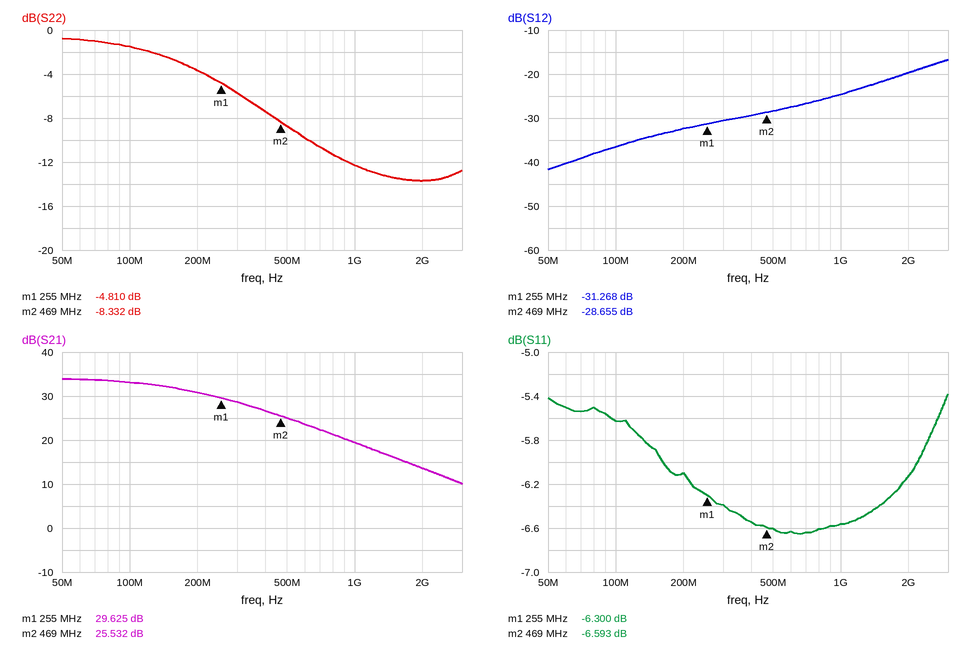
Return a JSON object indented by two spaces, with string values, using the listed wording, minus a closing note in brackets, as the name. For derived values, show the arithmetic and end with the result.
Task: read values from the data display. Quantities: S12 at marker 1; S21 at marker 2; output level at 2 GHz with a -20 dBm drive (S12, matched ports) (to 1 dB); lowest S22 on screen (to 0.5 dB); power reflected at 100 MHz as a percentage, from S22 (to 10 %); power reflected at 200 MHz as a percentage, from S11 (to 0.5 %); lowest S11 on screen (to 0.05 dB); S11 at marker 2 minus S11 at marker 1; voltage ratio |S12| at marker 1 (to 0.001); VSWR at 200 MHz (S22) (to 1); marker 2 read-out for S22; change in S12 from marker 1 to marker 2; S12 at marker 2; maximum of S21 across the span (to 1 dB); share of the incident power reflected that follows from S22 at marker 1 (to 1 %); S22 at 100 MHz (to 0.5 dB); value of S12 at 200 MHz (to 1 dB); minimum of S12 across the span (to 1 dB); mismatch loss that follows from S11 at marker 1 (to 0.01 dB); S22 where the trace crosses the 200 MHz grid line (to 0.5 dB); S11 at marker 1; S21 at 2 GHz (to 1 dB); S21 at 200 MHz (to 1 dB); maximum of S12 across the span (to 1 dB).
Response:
{
  "S12 at marker 1": "-31.268 dB",
  "S21 at marker 2": "25.532 dB",
  "output level at 2 GHz with a -20 dBm drive (S12, matched ports)": "-20 dBm + (-20 dB) = -40 dBm",
  "lowest S22 on screen": "-13.5 dB",
  "power reflected at 100 MHz as a percentage, from S22": "10^(-1.5/10) ≈ 70.8 %, so 70 % to the nearest 10 %",
  "power reflected at 200 MHz as a percentage, from S11": "10^(-6.1/10) ≈ 24.5 %",
  "lowest S11 on screen": "-6.65 dB",
  "S11 at marker 2 minus S11 at marker 1": "-6.593 − (-6.3) = -0.293 dB",
  "voltage ratio |S12| at marker 1": "10^(-31.268/20) ≈ 0.027",
  "VSWR at 200 MHz (S22)": "|Γ| = 10^(-3.5/20) = 0.6683; VSWR = (1 + 0.6683)/(1 − 0.6683) ≈ 5",
  "marker 2 read-out for S22": "-8.332 dB",
  "change in S12 from marker 1 to marker 2": "-28.655 − (-31.268) = 2.613 dB",
  "S12 at marker 2": "-28.655 dB",
  "maximum of S21 across the span": "34 dB",
  "share of the incident power reflected that follows from S22 at marker 1": "10^(-4.81/10) ≈ 33 %",
  "S22 at 100 MHz": "-1.5 dB",
  "value of S12 at 200 MHz": "-32 dB",
  "minimum of S12 across the span": "-42 dB",
  "mismatch loss that follows from S11 at marker 1": "−10 log10(1 − 10^(-6.3/10)) ≈ 1.16 dB",
  "S22 where the trace crosses the 200 MHz grid line": "-3.5 dB",
  "S11 at marker 1": "-6.300 dB",
  "S21 at 2 GHz": "14 dB",
  "S21 at 200 MHz": "31 dB",
  "maximum of S12 across the span": "-17 dB"
}
